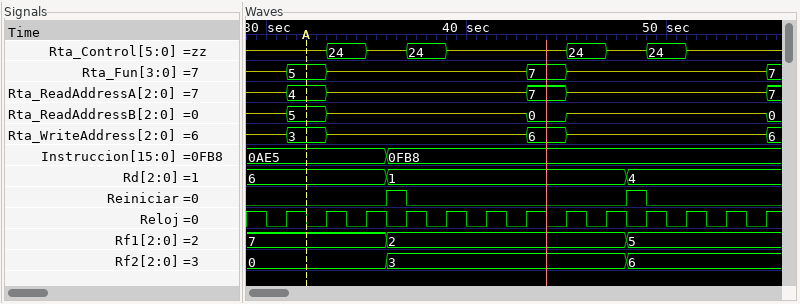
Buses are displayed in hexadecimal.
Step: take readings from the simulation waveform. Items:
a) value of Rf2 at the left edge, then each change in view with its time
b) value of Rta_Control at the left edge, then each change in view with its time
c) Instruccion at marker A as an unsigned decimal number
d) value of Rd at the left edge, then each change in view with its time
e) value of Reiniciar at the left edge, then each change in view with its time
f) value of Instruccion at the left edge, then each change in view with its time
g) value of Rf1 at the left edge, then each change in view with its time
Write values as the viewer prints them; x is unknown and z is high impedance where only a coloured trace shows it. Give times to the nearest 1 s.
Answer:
0, 3 at 36 s, 6 at 48 s
z, 24 at 33 s, z at 35 s, 24 at 37 s, z at 39 s, 24 at 45 s, z at 47 s, 24 at 49 s, z at 51 s
2789
6, 1 at 36 s, 4 at 48 s
0, 1 at 36 s, 0 at 37 s, 1 at 48 s, 0 at 49 s
0AE5, 0FB8 at 36 s
7, 2 at 36 s, 5 at 48 s
